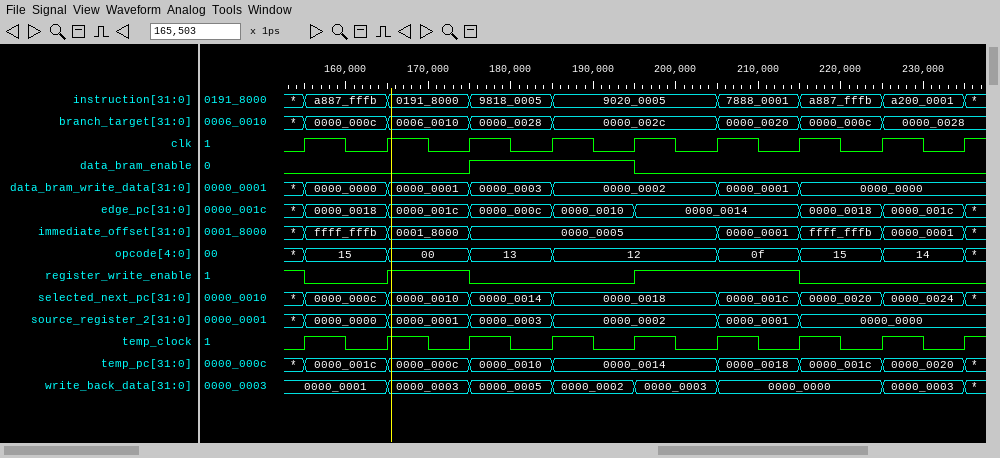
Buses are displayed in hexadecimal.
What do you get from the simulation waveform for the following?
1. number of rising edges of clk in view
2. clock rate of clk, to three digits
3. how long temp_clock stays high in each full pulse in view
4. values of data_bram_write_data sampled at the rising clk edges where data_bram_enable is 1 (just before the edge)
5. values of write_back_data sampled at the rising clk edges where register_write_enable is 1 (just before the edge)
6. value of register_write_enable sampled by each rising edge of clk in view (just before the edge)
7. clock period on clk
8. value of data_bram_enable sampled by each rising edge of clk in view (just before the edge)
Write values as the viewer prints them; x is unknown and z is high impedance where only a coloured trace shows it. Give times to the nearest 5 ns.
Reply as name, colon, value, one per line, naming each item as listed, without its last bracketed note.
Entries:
number of rising edges of clk in view: 9
clock rate of clk, to three digits: 100 MHz
how long temp_clock stays high in each full pulse in view: 5 ns, 5 ns, 5 ns, 5 ns, 5 ns, 5 ns, 5 ns, 5 ns
values of data_bram_write_data sampled at the rising clk edges where data_bram_enable is 1: 0000_0003, 0000_0002
values of write_back_data sampled at the rising clk edges where register_write_enable is 1: 0000_0001, 0000_0003, 0000_0003, 0000_0000
value of register_write_enable sampled by each rising edge of clk in view: 1 0 1 0 0 1 1 0 0
clock period on clk: 10 ns
value of data_bram_enable sampled by each rising edge of clk in view: 0 0 0 1 1 0 0 0 0
